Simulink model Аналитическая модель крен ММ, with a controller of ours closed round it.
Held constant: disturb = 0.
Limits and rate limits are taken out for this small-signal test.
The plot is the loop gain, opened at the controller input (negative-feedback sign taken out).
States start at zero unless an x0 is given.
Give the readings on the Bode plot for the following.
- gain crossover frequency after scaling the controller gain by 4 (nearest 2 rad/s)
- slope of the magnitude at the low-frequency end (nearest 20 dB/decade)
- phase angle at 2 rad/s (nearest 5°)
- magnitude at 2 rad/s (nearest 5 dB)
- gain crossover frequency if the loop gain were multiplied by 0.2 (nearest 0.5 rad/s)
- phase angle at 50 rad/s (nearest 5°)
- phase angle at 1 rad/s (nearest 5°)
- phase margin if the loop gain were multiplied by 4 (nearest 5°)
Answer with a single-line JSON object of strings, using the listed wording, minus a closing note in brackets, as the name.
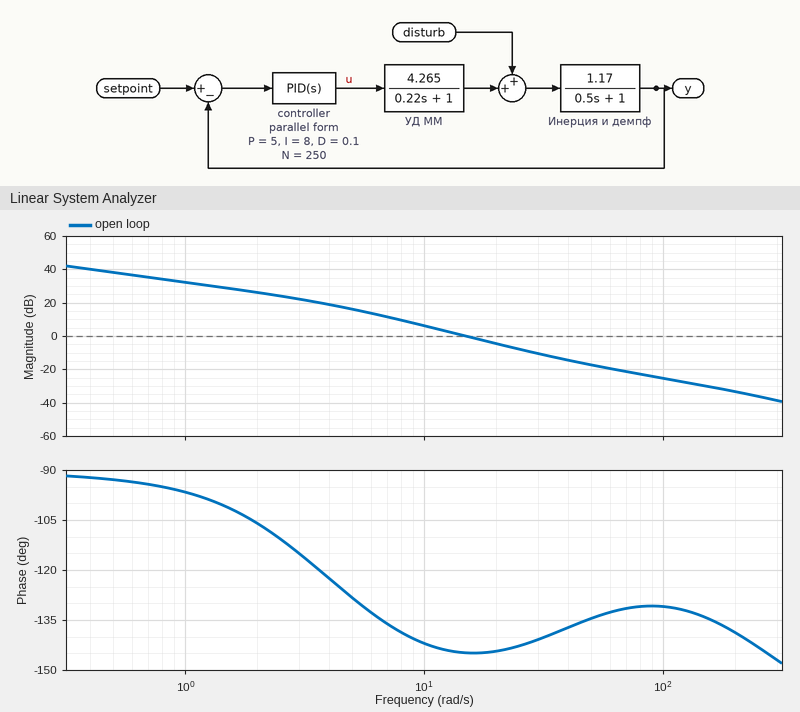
{"gain crossover frequency after scaling the controller gain by 4": "34 rad/s", "slope of the magnitude at the low-frequency end": "-20 dB/decade", "phase angle at 2 rad/s": "-105°", "magnitude at 2 rad/s": "25 dB", "gain crossover frequency if the loop gain were multiplied by 0.2": "6.0 rad/s", "phase angle at 50 rad/s": "-135°", "phase angle at 1 rad/s": "-95°", "phase margin if the loop gain were multiplied by 4": "40°"}
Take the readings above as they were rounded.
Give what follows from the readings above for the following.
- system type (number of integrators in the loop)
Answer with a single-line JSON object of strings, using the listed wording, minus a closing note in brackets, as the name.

{"system type": "1"}
